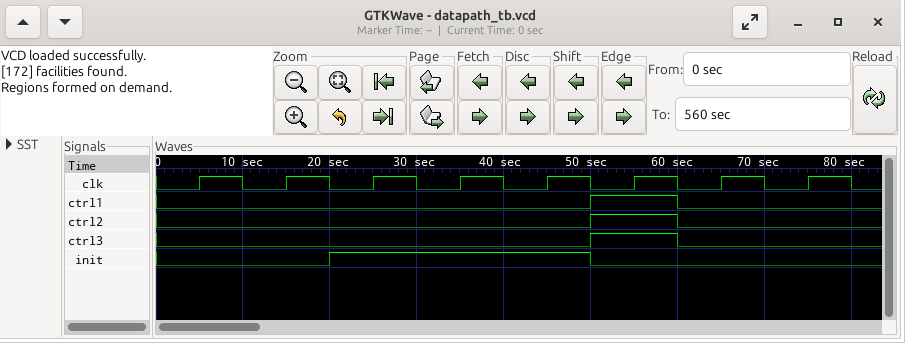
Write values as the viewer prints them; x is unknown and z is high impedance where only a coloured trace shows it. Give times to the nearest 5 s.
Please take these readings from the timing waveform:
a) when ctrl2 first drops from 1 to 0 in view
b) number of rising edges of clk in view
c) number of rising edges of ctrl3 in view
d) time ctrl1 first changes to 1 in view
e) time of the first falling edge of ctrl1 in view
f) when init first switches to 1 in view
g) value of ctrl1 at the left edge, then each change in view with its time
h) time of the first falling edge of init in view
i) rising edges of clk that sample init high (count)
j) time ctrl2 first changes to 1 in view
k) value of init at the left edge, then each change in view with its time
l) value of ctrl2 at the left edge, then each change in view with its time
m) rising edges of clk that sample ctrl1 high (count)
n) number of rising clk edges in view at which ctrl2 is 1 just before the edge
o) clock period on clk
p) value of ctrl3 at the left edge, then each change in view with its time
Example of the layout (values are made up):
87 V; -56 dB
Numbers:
60 s; 8; 1; 50 s; 60 s; 20 s; 0, 1 at 50 s, 0 at 60 s; 50 s; 3; 50 s; 0, 1 at 20 s, 0 at 50 s; 0, 1 at 50 s, 0 at 60 s; 1; 1; 10 s; 0, 1 at 50 s, 0 at 60 s
